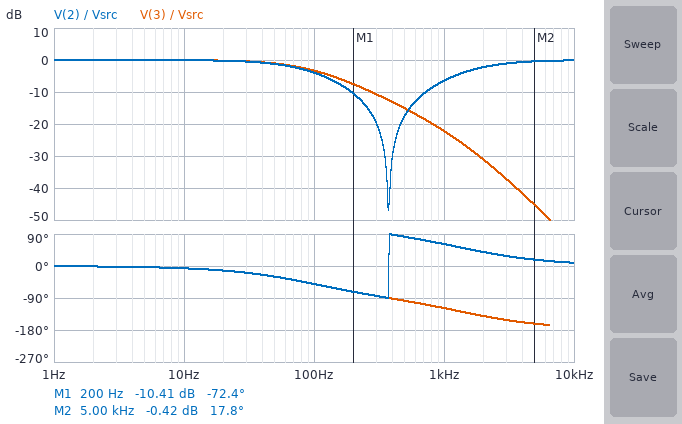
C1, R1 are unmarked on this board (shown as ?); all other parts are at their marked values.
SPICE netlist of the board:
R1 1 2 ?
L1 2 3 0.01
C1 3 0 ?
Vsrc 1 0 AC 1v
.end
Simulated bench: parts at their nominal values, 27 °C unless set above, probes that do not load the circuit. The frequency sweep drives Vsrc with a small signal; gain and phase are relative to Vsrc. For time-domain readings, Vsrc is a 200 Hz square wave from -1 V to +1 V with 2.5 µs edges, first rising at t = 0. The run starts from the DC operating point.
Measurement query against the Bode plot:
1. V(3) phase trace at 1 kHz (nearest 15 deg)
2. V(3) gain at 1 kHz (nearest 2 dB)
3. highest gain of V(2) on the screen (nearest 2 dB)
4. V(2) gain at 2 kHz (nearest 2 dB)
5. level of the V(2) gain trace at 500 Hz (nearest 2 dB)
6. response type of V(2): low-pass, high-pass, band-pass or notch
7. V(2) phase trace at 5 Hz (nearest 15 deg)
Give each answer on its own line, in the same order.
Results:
-120 deg
-22 dB
0 dB
-2 dB
-18 dB
notch
0 deg
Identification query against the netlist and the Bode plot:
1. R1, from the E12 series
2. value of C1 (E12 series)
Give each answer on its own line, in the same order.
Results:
100 Ω
18 µF
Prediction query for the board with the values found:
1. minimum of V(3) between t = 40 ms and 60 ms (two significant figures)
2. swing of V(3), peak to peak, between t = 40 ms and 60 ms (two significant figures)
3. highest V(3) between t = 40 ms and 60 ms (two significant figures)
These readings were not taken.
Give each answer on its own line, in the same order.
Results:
-610 mV
1.2 V
610 mV
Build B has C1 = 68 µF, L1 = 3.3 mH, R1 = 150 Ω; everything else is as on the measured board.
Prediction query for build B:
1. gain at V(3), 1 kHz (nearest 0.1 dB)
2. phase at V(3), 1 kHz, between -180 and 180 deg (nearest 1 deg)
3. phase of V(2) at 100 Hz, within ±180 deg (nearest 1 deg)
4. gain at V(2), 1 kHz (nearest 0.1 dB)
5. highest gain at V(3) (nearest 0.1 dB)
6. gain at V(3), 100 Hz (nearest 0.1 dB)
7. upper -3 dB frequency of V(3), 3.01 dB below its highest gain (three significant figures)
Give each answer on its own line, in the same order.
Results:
-36.2 dB
-97 deg
-82 deg
-18.3 dB
0 dB
-16.2 dB
15.6 Hz
